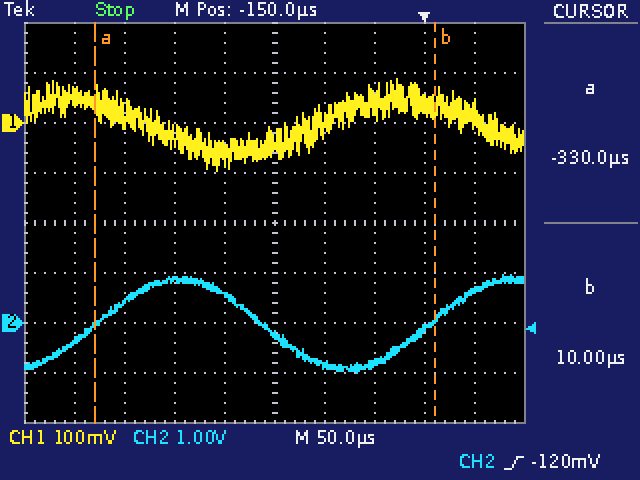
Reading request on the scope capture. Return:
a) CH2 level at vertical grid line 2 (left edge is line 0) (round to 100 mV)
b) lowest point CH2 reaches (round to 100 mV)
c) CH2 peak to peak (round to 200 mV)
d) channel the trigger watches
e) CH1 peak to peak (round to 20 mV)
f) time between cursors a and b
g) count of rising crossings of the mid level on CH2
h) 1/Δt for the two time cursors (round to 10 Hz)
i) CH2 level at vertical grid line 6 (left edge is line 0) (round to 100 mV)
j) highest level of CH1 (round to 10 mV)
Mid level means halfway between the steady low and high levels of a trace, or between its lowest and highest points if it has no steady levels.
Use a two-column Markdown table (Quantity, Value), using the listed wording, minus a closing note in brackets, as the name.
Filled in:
| Quantity | Value |
|---|---|
| CH2 level at vertical grid line 2 (left edge is line 0) | 400 mV |
| lowest point CH2 reaches | -1.0 V |
| CH2 peak to peak | 2.0 V |
| channel the trigger watches | CH2 |
| CH1 peak to peak | 180 mV |
| time between cursors a and b | 340 µs |
| count of rising crossings of the mid level on CH2 | 2 |
| 1/Δt for the two time cursors | 2.94 kHz |
| CH2 level at vertical grid line 6 (left edge is line 0) | -800 mV |
| highest level of CH1 | 90 mV |
